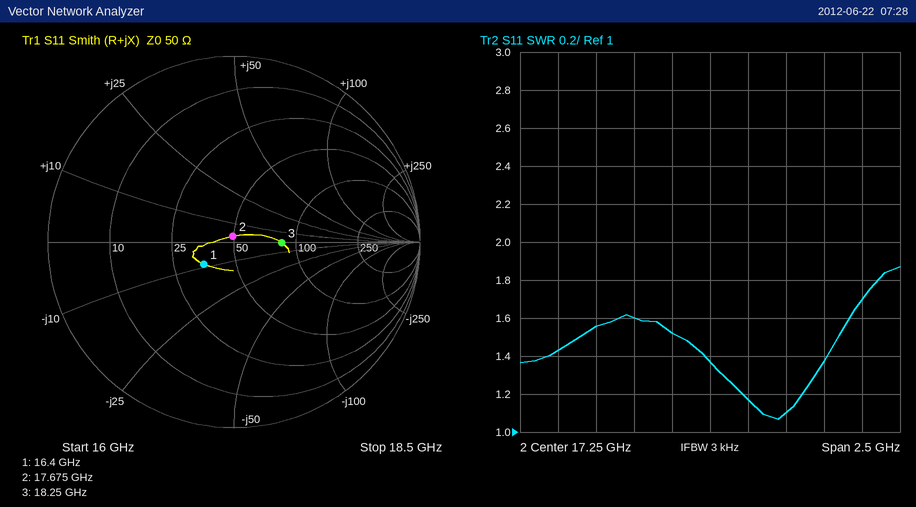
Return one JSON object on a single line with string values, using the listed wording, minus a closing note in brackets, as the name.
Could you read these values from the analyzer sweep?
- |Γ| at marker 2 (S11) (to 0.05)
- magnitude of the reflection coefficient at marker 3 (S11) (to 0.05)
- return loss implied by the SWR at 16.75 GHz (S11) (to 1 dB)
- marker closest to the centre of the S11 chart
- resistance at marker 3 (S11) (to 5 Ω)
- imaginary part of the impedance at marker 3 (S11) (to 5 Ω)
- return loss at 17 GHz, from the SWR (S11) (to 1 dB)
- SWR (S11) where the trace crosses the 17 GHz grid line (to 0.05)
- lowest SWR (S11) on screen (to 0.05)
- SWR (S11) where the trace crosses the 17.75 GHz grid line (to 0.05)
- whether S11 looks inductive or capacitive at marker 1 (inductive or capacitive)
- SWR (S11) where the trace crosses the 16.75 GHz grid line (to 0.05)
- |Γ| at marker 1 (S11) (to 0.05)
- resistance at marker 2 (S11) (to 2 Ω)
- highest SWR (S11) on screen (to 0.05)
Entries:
{"|Γ| at marker 2 (S11)": "0.05", "magnitude of the reflection coefficient at marker 3 (S11)": "0.25", "return loss implied by the SWR at 16.75 GHz (S11)": "13 dB", "marker closest to the centre of the S11 chart": "marker 2", "resistance at marker 3 (S11)": "85 Ω", "imaginary part of the impedance at marker 3 (S11)": "0 Ω", "return loss at 17 GHz, from the SWR (S11)": "14 dB", "SWR (S11) where the trace crosses the 17 GHz grid line": "1.50", "lowest SWR (S11) on screen": "1.05", "SWR (S11) where the trace crosses the 17.75 GHz grid line": "1.10", "whether S11 looks inductive or capacitive at marker 1": "capacitive", "SWR (S11) where the trace crosses the 16.75 GHz grid line": "1.60", "|Γ| at marker 1 (S11)": "0.20", "resistance at marker 2 (S11)": "50 Ω", "highest SWR (S11) on screen": "1.85"}
